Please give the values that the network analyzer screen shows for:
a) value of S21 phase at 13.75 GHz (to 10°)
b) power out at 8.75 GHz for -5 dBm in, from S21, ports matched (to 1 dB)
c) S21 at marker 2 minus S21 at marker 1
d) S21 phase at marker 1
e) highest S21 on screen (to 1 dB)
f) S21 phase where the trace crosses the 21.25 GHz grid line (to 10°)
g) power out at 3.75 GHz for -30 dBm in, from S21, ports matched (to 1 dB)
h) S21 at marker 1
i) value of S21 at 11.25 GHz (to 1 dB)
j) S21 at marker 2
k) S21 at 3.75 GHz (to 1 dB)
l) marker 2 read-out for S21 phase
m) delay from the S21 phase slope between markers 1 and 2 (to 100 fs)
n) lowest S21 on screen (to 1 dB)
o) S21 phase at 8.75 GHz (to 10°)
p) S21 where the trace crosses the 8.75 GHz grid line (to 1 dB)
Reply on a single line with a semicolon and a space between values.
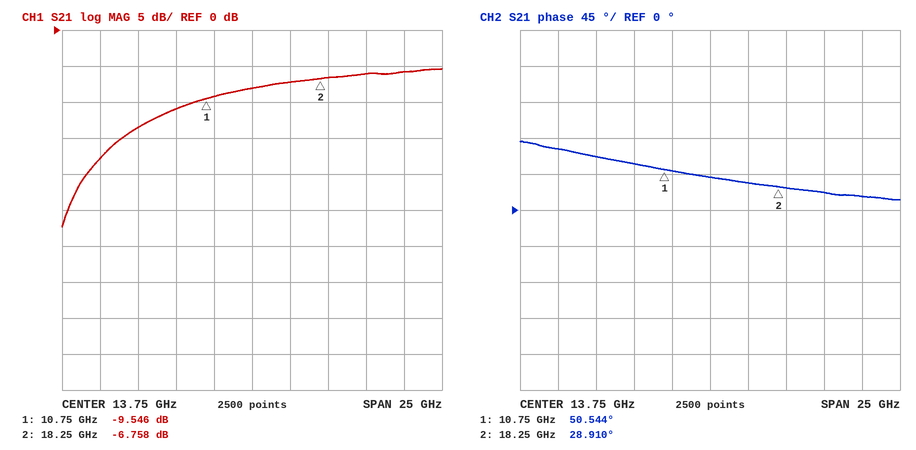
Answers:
40°; -16 dBm; 2.788 dB; 50.544°; -5 dB; 20°; -48 dBm; -9.546 dB; -9 dB; -6.758 dB; -18 dB; 28.910°; 8.0 ps; -27 dB; 60°; -11 dB
